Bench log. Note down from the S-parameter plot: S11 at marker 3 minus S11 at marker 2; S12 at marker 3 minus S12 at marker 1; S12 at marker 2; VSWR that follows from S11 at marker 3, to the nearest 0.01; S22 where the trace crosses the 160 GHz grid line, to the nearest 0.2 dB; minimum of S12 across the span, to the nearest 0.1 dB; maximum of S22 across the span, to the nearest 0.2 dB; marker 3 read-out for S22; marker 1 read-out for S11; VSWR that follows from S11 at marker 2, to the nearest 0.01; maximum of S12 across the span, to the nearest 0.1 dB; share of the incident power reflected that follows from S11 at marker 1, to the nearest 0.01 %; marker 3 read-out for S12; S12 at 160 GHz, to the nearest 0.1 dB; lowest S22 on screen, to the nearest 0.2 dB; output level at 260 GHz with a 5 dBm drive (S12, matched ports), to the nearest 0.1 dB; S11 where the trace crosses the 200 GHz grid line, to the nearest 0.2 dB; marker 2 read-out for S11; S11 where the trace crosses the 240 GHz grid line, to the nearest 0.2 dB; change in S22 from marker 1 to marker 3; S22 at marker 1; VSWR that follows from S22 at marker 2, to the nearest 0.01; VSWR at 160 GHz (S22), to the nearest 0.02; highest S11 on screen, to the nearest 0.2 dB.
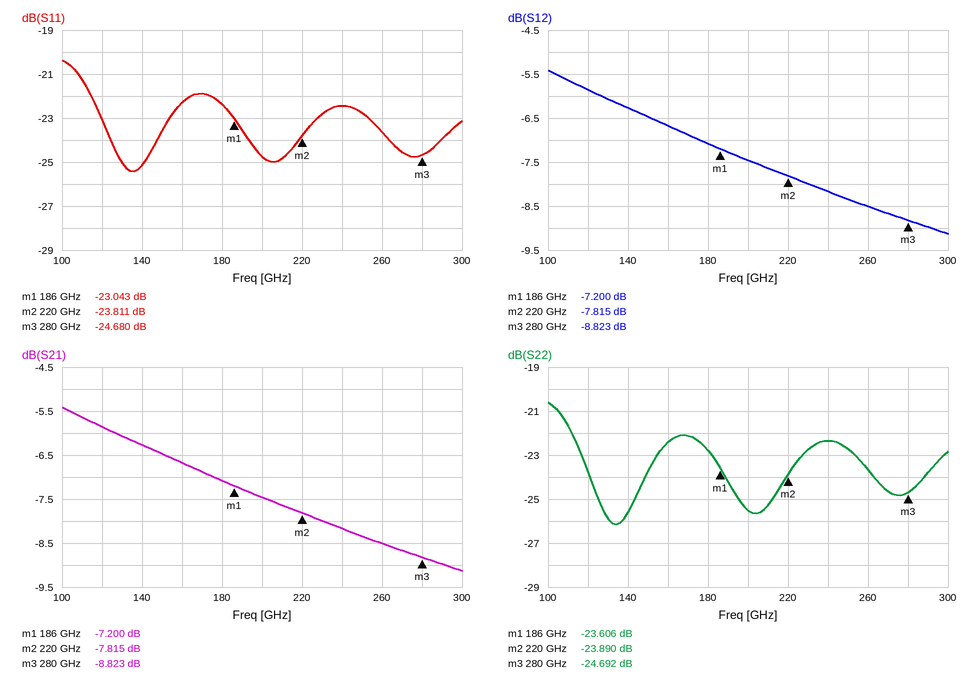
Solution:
-0.869 dB
-1.623 dB
-7.815 dB
1.12
-22.4 dB
-9.1 dB
-20.6 dB
-24.692 dB
-23.043 dB
1.14
-5.4 dB
0.50 %
-8.823 dB
-6.7 dB
-26.2 dB
-3.5 dBm
-24.8 dB
-23.811 dB
-22.4 dB
-1.086 dB
-23.606 dB
1.14
1.16
-20.4 dB
